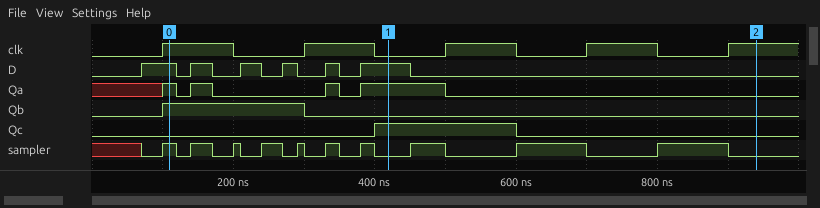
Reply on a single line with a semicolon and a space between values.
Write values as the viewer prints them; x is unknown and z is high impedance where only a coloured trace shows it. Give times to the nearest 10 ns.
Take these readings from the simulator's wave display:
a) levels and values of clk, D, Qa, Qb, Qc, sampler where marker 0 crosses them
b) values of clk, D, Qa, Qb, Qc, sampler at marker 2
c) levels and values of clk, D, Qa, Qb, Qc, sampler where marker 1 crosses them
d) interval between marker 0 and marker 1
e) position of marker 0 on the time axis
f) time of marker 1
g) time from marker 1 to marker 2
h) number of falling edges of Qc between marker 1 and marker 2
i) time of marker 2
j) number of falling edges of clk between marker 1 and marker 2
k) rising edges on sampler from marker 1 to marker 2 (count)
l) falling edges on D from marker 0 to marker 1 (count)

clk=1, D=1, Qa=1, Qb=1, Qc=0, sampler=1; clk=1, D=0, Qa=0, Qb=0, Qc=0, sampler=0; clk=0, D=1, Qa=1, Qb=0, Qc=1, sampler=0; 310 ns; 110 ns; 420 ns; 520 ns; 1; 940 ns; 2; 3; 5
